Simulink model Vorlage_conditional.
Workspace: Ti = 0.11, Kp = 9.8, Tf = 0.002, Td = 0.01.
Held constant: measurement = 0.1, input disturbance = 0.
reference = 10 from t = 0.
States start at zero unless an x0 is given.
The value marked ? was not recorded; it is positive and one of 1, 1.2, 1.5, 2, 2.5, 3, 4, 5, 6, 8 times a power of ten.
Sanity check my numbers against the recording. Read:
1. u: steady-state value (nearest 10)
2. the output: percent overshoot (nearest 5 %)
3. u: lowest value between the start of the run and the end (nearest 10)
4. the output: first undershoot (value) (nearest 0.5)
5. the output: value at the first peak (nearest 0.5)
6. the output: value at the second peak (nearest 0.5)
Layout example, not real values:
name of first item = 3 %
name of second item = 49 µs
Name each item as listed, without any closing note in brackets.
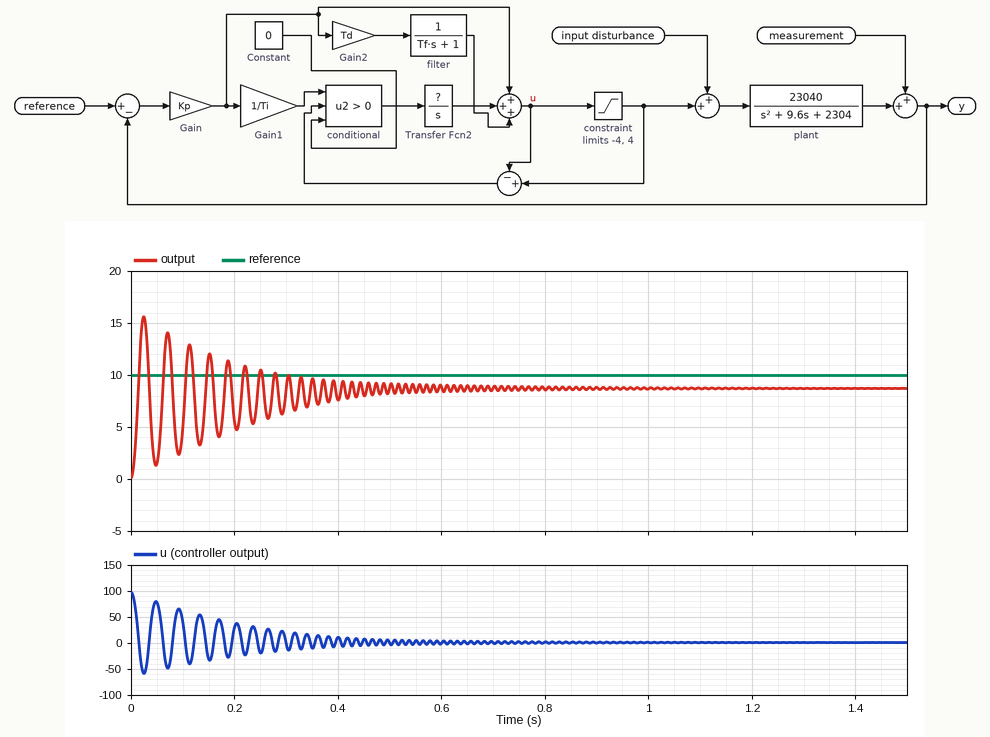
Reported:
u: steady-state value = 0
the output: percent overshoot = 80 %
u: lowest value between the start of the run and the end = -60
the output: first undershoot (value) = 1.5
the output: value at the first peak = 15.5
the output: value at the second peak = 14.0
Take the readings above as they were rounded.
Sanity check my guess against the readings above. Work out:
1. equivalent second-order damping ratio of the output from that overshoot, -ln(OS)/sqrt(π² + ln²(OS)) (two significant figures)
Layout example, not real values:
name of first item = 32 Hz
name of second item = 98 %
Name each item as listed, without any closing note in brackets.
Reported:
equivalent second-order damping ratio of the output from that overshoot, -ln(OS)/sqrt(π² + ln²(OS)) = 0.071
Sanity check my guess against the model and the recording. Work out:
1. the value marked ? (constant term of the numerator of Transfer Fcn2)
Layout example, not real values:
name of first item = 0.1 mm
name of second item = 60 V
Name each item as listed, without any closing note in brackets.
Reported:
the value marked ? = 1
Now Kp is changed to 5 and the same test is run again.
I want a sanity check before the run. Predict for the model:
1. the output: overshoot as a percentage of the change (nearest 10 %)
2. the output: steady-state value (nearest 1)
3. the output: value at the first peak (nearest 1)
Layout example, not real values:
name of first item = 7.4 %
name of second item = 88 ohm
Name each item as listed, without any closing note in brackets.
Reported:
the output: overshoot as a percentage of the change = 90 %
the output: steady-state value = 8
the output: value at the first peak = 16
